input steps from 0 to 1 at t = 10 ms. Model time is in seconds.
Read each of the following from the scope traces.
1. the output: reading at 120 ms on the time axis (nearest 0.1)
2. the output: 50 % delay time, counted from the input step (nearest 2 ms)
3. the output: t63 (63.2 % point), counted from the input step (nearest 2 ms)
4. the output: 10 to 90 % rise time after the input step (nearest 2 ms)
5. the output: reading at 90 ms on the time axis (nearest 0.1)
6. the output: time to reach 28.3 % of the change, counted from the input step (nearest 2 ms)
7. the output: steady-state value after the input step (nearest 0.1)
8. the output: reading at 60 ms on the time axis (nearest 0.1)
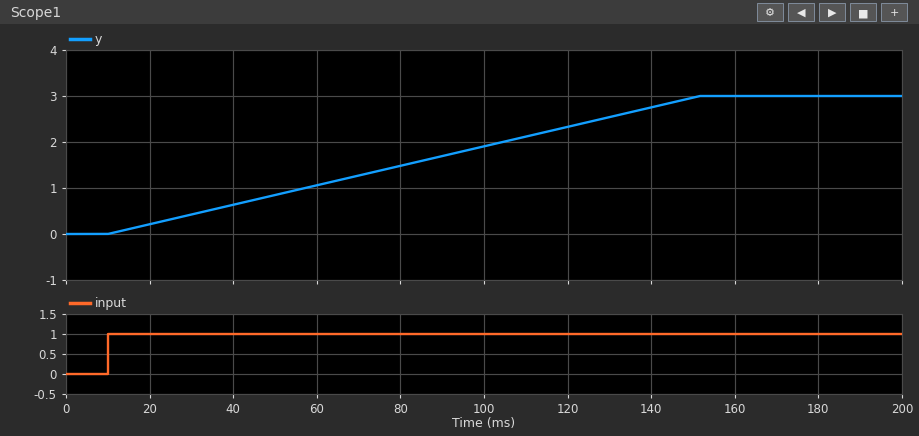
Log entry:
2.3
70 ms
90 ms
114 ms
1.7
40 ms
3.0
1.1
